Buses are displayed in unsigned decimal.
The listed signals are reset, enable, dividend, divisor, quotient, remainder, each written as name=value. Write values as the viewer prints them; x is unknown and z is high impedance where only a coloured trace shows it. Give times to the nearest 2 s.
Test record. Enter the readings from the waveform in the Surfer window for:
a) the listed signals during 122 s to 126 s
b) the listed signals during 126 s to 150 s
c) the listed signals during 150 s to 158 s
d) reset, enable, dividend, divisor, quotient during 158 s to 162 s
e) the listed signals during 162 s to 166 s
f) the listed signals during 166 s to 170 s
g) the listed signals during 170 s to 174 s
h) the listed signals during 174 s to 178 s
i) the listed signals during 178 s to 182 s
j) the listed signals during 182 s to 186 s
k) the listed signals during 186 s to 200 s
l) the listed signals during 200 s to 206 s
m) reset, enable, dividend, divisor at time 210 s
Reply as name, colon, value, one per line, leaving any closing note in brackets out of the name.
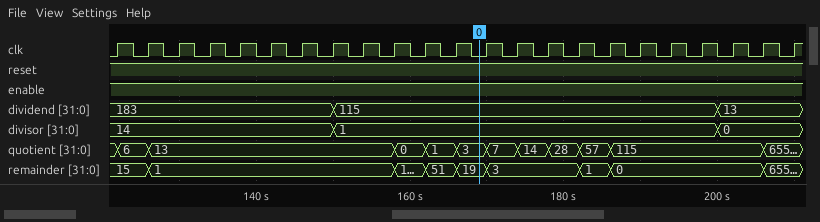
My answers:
the listed signals during 122 s to 126 s: reset=1, enable=1, dividend=183, divisor=14, quotient=6, remainder=15
the listed signals during 126 s to 150 s: reset=1, enable=1, dividend=183, divisor=14, quotient=13, remainder=1
the listed signals during 150 s to 158 s: reset=1, enable=1, dividend=115, divisor=1, quotient=13, remainder=1
reset, enable, dividend, divisor, quotient during 158 s to 162 s: reset=1, enable=1, dividend=115, divisor=1, quotient=0
the listed signals during 162 s to 166 s: reset=1, enable=1, dividend=115, divisor=1, quotient=1, remainder=51
the listed signals during 166 s to 170 s: reset=1, enable=1, dividend=115, divisor=1, quotient=3, remainder=19
the listed signals during 170 s to 174 s: reset=1, enable=1, dividend=115, divisor=1, quotient=7, remainder=3
the listed signals during 174 s to 178 s: reset=1, enable=1, dividend=115, divisor=1, quotient=14, remainder=3
the listed signals during 178 s to 182 s: reset=1, enable=1, dividend=115, divisor=1, quotient=28, remainder=3
the listed signals during 182 s to 186 s: reset=1, enable=1, dividend=115, divisor=1, quotient=57, remainder=1
the listed signals during 186 s to 200 s: reset=1, enable=1, dividend=115, divisor=1, quotient=115, remainder=0
the listed signals during 200 s to 206 s: reset=1, enable=1, dividend=13, divisor=0, quotient=115, remainder=0
reset, enable, dividend, divisor at time 210 s: reset=1, enable=1, dividend=13, divisor=0
